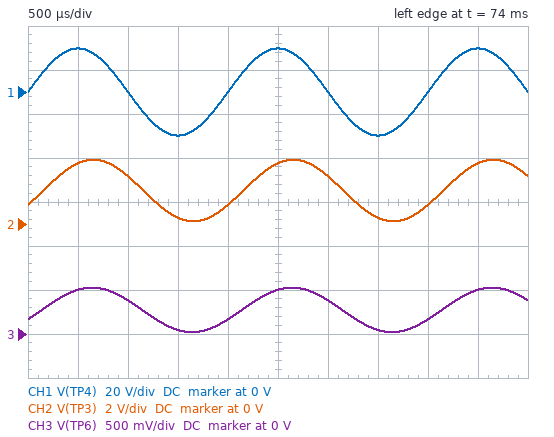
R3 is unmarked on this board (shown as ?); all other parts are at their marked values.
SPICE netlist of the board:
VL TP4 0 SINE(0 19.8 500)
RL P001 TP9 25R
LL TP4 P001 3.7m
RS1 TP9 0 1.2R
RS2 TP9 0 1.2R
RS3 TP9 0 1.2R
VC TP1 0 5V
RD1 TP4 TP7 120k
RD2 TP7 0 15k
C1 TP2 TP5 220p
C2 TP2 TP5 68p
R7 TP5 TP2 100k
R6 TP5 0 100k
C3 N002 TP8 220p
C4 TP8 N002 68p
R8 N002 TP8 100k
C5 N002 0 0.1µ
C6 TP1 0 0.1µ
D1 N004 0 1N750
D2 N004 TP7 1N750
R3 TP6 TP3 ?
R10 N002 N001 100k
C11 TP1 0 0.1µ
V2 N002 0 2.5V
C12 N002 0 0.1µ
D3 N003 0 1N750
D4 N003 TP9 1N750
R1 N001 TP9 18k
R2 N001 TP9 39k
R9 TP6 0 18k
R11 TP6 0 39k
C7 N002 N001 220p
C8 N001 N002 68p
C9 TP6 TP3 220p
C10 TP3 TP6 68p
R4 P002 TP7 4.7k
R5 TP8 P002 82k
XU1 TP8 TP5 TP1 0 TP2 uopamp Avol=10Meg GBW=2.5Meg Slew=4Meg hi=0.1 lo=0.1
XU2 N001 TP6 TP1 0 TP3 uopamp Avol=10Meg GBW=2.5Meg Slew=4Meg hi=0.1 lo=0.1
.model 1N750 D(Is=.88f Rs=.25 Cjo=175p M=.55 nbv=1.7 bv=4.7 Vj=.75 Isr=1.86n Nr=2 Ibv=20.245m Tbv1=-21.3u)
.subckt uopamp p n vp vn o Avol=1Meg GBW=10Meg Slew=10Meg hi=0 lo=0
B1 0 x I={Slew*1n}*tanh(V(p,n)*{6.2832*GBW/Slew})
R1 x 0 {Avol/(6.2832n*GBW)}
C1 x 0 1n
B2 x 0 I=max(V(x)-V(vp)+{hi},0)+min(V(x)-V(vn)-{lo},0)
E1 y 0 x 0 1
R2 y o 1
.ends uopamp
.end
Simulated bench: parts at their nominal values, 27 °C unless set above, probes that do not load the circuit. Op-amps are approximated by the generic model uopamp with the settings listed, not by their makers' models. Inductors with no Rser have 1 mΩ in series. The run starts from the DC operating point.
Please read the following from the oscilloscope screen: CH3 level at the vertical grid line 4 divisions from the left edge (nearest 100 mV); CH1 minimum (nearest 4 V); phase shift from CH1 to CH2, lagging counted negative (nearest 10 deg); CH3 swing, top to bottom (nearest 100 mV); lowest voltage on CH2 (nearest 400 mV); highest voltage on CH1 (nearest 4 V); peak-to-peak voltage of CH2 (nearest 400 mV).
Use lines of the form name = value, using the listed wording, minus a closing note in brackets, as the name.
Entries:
CH3 level at the vertical grid line 4 divisions from the left edge = 200 mV
CH1 minimum = -20 V
phase shift from CH1 to CH2, lagging counted negative = -30 deg
CH3 swing, top to bottom = 500 mV
lowest voltage on CH2 = 0 V
highest voltage on CH1 = 20 V
peak-to-peak voltage of CH2 = 2.8 V
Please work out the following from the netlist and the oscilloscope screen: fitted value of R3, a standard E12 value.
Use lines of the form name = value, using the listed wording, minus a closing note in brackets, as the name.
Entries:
fitted value of R3, a standard E12 value = 56 kΩ
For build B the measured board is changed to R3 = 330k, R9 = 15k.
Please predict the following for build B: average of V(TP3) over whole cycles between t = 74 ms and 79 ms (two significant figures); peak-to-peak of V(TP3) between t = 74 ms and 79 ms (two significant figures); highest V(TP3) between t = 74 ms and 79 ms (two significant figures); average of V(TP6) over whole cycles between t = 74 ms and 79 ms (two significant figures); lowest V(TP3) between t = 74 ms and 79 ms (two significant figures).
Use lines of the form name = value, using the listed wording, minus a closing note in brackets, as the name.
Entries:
average of V(TP3) over whole cycles between t = 74 ms and 79 ms = 4.0 V
peak-to-peak of V(TP3) between t = 74 ms and 79 ms = 3.9 V
highest V(TP3) between t = 74 ms and 79 ms = 4.9 V
average of V(TP6) over whole cycles between t = 74 ms and 79 ms = 130 mV
lowest V(TP3) between t = 74 ms and 79 ms = 1.0 V
